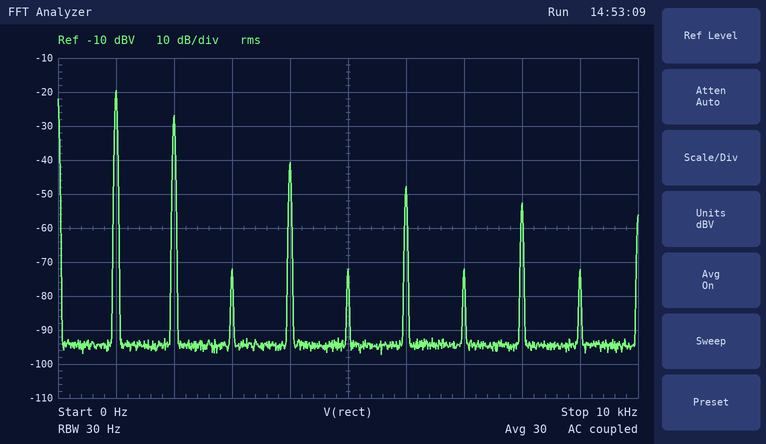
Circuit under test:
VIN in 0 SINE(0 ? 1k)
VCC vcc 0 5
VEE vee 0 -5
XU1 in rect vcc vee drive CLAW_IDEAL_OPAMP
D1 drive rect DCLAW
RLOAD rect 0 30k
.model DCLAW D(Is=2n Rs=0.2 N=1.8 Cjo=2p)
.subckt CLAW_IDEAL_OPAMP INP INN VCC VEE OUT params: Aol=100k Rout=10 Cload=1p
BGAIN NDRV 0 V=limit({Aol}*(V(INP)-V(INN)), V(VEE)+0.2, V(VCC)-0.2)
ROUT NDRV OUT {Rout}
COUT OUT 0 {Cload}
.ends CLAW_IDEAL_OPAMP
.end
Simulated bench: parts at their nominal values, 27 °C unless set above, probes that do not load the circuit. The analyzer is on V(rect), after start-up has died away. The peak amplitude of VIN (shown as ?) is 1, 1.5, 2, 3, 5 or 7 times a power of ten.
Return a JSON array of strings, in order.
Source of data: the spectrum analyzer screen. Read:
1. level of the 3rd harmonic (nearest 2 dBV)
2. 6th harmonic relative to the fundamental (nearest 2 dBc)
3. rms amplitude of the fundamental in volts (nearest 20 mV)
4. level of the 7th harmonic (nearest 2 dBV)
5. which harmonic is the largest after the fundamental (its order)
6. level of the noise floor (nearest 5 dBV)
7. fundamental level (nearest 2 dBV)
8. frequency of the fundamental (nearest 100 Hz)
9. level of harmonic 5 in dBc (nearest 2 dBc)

["-72 dBV", "-28 dBc", "100 mV", "-72 dBV", "2", "-95 dBV", "-20 dBV", "1.0 kHz", "-52 dBc"]
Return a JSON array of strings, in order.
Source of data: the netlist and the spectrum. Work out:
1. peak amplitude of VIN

["300 mV"]
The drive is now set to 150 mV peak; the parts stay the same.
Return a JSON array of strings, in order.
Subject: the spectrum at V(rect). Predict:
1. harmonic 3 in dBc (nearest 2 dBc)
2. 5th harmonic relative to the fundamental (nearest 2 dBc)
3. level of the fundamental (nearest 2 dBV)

["-46 dBc", "-46 dBc", "-26 dBV"]
